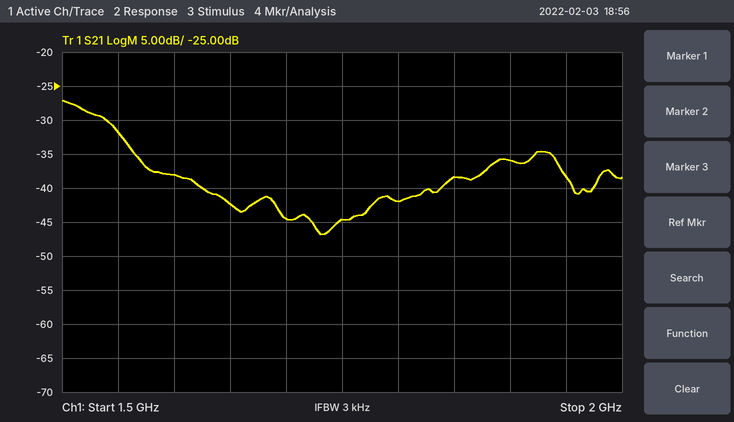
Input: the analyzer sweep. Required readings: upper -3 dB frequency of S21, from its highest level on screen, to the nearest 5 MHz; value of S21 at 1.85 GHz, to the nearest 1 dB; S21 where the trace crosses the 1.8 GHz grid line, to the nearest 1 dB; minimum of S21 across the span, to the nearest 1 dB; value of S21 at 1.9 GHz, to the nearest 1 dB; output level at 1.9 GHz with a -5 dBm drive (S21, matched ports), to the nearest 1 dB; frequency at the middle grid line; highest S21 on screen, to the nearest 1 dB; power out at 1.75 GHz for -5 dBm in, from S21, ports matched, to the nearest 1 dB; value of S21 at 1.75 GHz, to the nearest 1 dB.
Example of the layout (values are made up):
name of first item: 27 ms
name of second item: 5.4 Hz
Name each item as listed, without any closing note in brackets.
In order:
upper -3 dB frequency of S21, from its highest level on screen, to the nearest 5 MHz: 1.540 GHz
value of S21 at 1.85 GHz, to the nearest 1 dB: -38 dB
S21 where the trace crosses the 1.8 GHz grid line, to the nearest 1 dB: -42 dB
minimum of S21 across the span, to the nearest 1 dB: -47 dB
value of S21 at 1.9 GHz, to the nearest 1 dB: -36 dB
output level at 1.9 GHz with a -5 dBm drive (S21, matched ports), to the nearest 1 dB: -41 dBm
frequency at the middle grid line: 1.75 GHz
highest S21 on screen, to the nearest 1 dB: -27 dB
power out at 1.75 GHz for -5 dBm in, from S21, ports matched, to the nearest 1 dB: -50 dBm
value of S21 at 1.75 GHz, to the nearest 1 dB: -45 dB
